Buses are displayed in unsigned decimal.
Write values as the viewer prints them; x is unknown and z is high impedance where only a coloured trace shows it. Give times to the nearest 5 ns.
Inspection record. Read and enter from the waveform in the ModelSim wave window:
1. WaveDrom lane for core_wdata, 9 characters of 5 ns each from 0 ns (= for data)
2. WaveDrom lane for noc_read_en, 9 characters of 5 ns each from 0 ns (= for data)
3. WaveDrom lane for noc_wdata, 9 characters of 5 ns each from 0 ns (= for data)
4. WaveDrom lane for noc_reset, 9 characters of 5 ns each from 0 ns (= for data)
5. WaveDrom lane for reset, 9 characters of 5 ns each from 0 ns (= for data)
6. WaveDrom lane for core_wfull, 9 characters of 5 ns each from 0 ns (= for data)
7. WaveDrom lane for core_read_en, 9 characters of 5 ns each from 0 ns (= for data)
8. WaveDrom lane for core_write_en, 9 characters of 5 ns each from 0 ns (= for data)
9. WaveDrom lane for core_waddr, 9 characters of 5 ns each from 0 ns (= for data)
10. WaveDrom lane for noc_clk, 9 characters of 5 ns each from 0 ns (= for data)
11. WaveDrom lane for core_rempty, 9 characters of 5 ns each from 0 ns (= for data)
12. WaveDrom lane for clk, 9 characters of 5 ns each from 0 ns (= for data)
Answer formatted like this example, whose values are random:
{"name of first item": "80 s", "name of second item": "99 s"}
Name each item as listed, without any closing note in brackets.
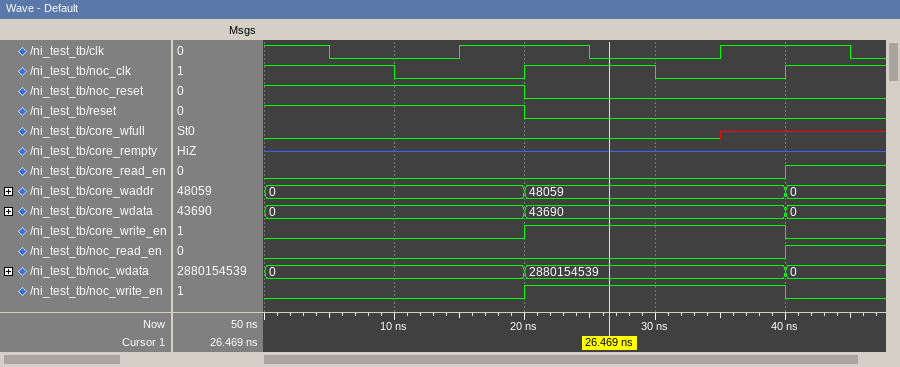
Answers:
{"WaveDrom lane for core_wdata, 9 characters of 5 ns each from 0 ns": "{name: 'core_wdata', wave: '=...=...=', data: '0 43690 0'}", "WaveDrom lane for noc_read_en, 9 characters of 5 ns each from 0 ns": "{name: 'noc_read_en', wave: '0.......1'}", "WaveDrom lane for noc_wdata, 9 characters of 5 ns each from 0 ns": "{name: 'noc_wdata', wave: '=...=...=', data: '0 2880154539 0'}", "WaveDrom lane for noc_reset, 9 characters of 5 ns each from 0 ns": "{name: 'noc_reset', wave: '1...0....'}", "WaveDrom lane for reset, 9 characters of 5 ns each from 0 ns": "{name: 'reset', wave: '1...0....'}", "WaveDrom lane for core_wfull, 9 characters of 5 ns each from 0 ns": "{name: 'core_wfull', wave: '0......x.'}", "WaveDrom lane for core_read_en, 9 characters of 5 ns each from 0 ns": "{name: 'core_read_en', wave: '0.......1'}", "WaveDrom lane for core_write_en, 9 characters of 5 ns each from 0 ns": "{name: 'core_write_en', wave: '0...1...0'}", "WaveDrom lane for core_waddr, 9 characters of 5 ns each from 0 ns": "{name: 'core_waddr', wave: '=...=...=', data: '0 48059 0'}", "WaveDrom lane for noc_clk, 9 characters of 5 ns each from 0 ns": "{name: 'noc_clk', wave: '1.0.1.0.1'}", "WaveDrom lane for core_rempty, 9 characters of 5 ns each from 0 ns": "{name: 'core_rempty', wave: 'z........'}", "WaveDrom lane for clk, 9 characters of 5 ns each from 0 ns": "{name: 'clk', wave: '10.1.0.1.'}"}
